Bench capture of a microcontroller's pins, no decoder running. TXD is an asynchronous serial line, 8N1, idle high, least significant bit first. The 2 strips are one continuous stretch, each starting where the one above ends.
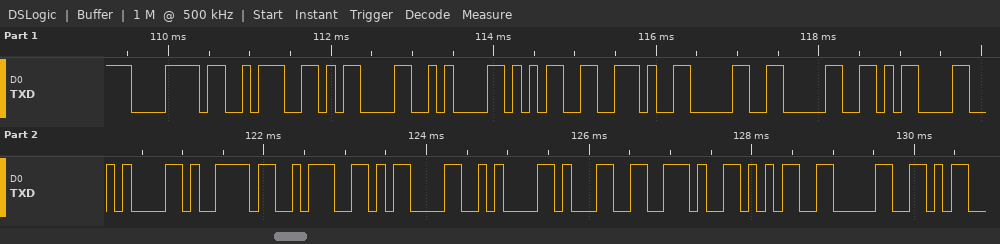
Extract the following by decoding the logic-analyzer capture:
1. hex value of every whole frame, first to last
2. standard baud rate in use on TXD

0x78 0x3A 0x0D 0x0A 0x35 0x2E 0x30 0x30 0x0D 0x0A 0x79 0x3A 0x0D 0x0A 0x31 0x2E 0x35 0x30
9600 baud
